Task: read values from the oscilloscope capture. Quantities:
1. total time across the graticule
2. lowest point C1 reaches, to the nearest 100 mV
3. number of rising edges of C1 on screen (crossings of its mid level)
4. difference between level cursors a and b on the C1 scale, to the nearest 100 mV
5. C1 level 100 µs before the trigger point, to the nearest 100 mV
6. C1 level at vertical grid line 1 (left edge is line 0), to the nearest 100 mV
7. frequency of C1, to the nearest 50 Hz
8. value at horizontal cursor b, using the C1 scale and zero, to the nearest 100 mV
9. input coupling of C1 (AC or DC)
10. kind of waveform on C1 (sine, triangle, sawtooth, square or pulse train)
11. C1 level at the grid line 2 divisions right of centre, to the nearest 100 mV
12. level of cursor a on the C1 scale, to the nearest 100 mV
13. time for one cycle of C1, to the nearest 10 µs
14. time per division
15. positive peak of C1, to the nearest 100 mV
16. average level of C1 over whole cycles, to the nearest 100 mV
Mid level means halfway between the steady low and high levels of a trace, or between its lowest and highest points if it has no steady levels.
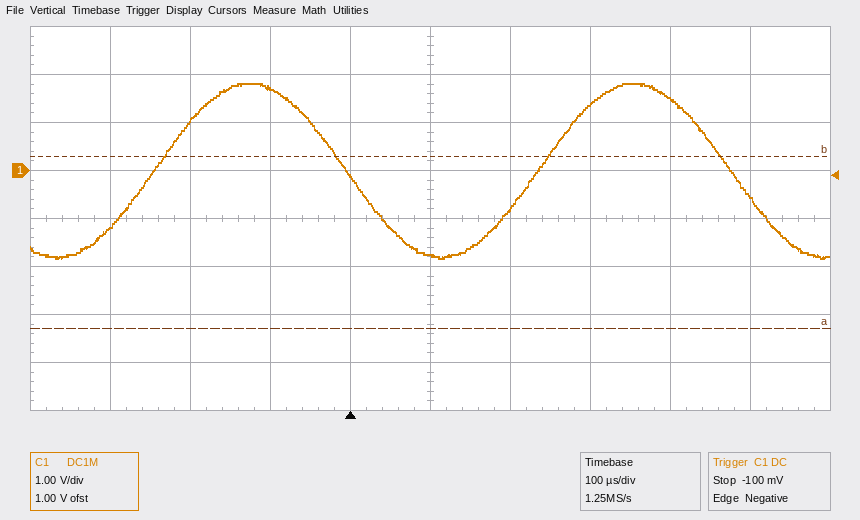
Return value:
1 ms
-1.8 V
2
3.6 V
1.7 V
-1.2 V
2.10 kHz
300 mV
DC
sine
1.4 V
-3.3 V
480 µs
100 µs
1.8 V
0.0 V
